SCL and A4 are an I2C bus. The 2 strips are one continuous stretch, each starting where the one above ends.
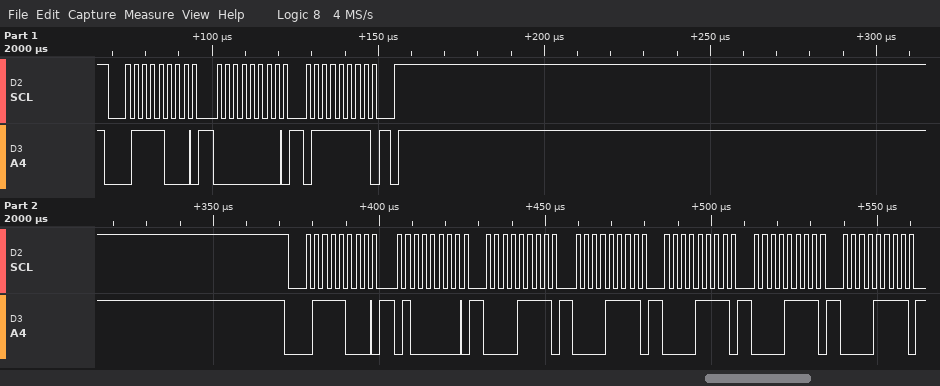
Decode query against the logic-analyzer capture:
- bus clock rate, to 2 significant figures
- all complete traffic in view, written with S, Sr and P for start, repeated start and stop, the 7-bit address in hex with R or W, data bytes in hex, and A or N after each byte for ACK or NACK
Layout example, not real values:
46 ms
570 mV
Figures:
400 kHz
S 3CW A 00 A 7F A P S 3CW A 40 A 0F A 0F A 0F A 0F A 0F A
